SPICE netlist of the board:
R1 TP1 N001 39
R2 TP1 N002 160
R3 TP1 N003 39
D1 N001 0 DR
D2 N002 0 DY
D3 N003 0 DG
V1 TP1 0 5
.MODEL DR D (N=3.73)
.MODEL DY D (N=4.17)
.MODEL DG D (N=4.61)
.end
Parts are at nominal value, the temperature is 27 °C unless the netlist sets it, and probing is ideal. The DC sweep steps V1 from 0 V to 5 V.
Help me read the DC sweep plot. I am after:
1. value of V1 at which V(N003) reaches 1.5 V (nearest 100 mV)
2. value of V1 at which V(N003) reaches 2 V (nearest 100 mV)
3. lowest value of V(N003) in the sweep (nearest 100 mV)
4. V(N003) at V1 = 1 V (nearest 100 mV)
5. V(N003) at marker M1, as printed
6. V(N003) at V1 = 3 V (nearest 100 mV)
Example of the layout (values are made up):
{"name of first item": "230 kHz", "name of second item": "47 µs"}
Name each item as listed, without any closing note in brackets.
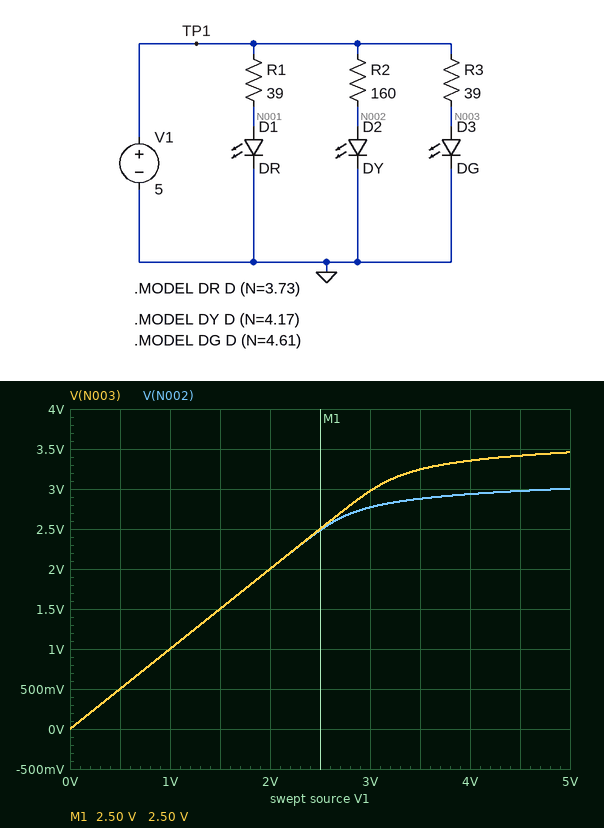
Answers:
{"value of V1 at which V(N003) reaches 1.5 V": "1.5 V", "value of V1 at which V(N003) reaches 2 V": "2.0 V", "lowest value of V(N003) in the sweep": "0 V", "V(N003) at V1 = 1 V": "1.0 V", "V(N003) at marker M1, as printed": "2.50 V", "V(N003) at V1 = 3 V": "3.0 V"}
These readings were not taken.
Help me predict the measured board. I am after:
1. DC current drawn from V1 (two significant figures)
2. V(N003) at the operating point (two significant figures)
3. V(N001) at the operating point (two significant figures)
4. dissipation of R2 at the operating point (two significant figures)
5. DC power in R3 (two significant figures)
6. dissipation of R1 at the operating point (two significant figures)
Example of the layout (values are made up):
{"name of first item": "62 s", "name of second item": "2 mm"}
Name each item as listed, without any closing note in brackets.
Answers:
{"DC current drawn from V1": "110 mA", "V(N003) at the operating point": "3.5 V", "V(N001) at the operating point": "2.8 V", "dissipation of R2 at the operating point": "25 mW", "DC power in R3": "61 mW", "dissipation of R1 at the operating point": "120 mW"}
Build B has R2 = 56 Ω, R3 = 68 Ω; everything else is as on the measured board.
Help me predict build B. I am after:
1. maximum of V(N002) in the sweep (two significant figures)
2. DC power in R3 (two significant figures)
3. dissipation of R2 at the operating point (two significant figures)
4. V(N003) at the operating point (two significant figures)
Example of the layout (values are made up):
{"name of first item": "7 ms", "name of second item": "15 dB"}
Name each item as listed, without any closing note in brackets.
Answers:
{"maximum of V(N002) in the sweep": "3.1 V", "DC power in R3": "38 mW", "dissipation of R2 at the operating point": "64 mW", "V(N003) at the operating point": "3.4 V"}
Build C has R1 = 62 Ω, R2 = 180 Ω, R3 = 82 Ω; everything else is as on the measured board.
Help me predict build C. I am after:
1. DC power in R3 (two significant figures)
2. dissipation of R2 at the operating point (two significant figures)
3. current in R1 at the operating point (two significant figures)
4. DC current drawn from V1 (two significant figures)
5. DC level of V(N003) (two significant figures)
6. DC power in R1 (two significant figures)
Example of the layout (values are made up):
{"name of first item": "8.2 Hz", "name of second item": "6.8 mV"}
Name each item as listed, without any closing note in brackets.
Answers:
{"DC power in R3": "32 mW", "dissipation of R2 at the operating point": "22 mW", "current in R1 at the operating point": "36 mA", "DC current drawn from V1": "67 mA", "DC level of V(N003)": "3.4 V", "DC power in R1": "79 mW"}
